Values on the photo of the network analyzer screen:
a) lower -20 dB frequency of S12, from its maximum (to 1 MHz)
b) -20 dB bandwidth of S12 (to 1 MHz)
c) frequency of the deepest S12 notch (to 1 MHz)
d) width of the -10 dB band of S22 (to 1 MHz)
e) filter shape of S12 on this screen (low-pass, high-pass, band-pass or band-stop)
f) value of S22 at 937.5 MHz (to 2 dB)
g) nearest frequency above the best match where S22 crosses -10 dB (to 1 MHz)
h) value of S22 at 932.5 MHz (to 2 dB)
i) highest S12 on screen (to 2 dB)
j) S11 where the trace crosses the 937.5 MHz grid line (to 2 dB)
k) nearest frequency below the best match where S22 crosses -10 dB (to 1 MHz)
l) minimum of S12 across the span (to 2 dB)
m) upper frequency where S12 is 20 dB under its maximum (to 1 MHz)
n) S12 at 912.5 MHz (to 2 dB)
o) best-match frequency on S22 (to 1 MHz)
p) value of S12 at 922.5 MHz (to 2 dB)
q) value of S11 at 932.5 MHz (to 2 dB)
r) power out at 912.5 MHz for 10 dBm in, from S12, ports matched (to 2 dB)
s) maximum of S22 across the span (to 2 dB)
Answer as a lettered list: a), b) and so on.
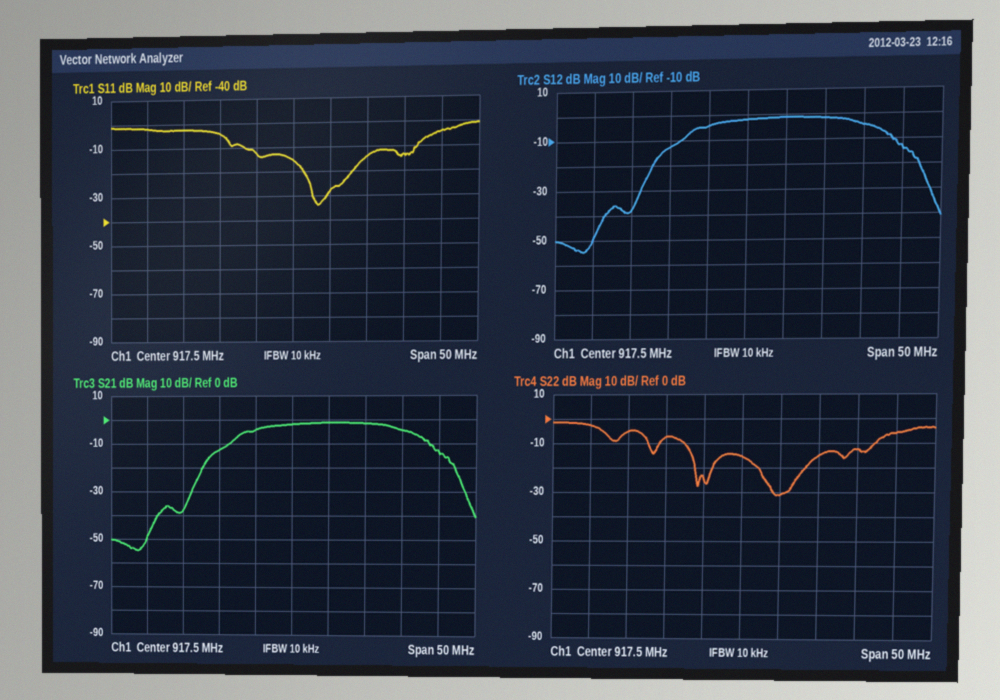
a) 905 MHz
b) 35 MHz
c) 896 MHz
d) 25 MHz
e) band-pass
f) -6 dB
g) 935 MHz
h) -12 dB
i) -2 dB
j) -4 dB
k) 910 MHz
l) -54 dB
m) 940 MHz
n) -4 dB
o) 922 MHz
p) -2 dB
q) -14 dB
r) 6 dBm
s) -2 dB
